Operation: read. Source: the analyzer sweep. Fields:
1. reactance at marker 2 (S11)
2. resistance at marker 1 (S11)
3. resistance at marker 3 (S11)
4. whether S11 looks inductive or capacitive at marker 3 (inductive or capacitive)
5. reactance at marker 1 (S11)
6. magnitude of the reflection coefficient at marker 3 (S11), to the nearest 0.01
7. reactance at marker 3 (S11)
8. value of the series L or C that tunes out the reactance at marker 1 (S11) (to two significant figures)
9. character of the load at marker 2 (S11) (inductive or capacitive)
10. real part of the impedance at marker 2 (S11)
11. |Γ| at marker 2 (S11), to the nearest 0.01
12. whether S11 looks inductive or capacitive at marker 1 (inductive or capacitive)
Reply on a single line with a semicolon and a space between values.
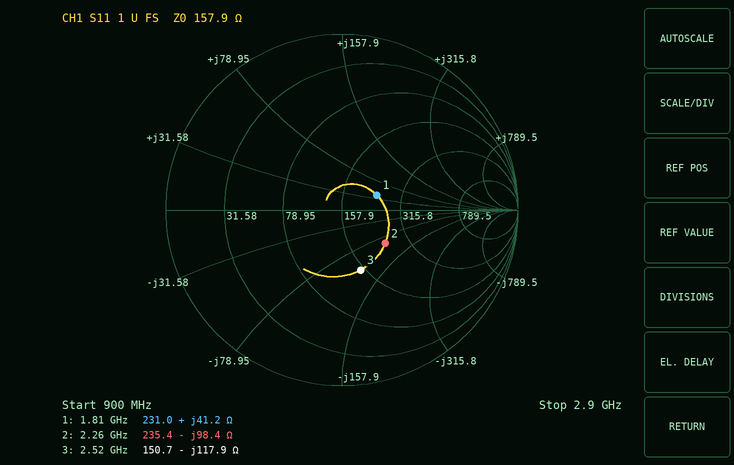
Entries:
-98.4 Ω; 231.0 Ω; 150.7 Ω; capacitive; +41.2 Ω; 0.36; -117.9 Ω; 2.1 pF; capacitive; 235.4 Ω; 0.31; inductive
